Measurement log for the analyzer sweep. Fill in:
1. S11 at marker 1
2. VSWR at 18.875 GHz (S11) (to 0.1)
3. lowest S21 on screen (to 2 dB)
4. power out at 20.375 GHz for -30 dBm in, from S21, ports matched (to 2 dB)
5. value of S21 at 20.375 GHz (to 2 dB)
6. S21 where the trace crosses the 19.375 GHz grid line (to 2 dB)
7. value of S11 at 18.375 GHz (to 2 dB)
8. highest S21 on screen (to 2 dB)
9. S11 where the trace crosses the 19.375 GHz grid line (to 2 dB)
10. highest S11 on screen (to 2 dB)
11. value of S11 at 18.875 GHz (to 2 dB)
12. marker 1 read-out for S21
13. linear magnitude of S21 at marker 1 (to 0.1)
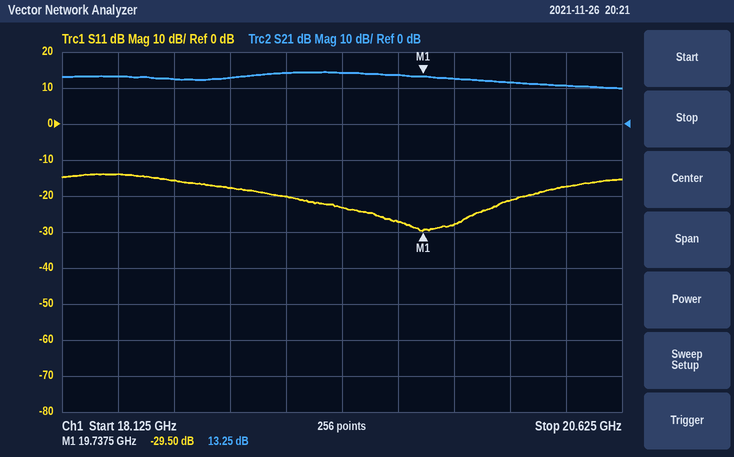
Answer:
-29.50 dB
1.3
10 dB
-20 dBm
10 dB
14 dB
-14 dB
14 dB
-24 dB
-14 dB
-18 dB
13.25 dB
4.6
